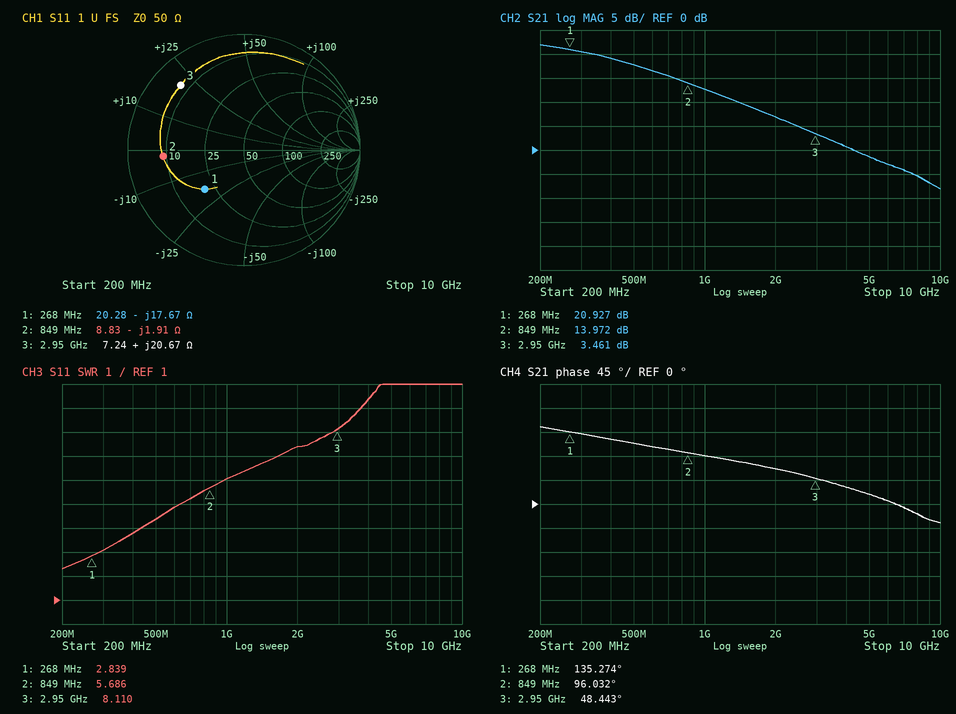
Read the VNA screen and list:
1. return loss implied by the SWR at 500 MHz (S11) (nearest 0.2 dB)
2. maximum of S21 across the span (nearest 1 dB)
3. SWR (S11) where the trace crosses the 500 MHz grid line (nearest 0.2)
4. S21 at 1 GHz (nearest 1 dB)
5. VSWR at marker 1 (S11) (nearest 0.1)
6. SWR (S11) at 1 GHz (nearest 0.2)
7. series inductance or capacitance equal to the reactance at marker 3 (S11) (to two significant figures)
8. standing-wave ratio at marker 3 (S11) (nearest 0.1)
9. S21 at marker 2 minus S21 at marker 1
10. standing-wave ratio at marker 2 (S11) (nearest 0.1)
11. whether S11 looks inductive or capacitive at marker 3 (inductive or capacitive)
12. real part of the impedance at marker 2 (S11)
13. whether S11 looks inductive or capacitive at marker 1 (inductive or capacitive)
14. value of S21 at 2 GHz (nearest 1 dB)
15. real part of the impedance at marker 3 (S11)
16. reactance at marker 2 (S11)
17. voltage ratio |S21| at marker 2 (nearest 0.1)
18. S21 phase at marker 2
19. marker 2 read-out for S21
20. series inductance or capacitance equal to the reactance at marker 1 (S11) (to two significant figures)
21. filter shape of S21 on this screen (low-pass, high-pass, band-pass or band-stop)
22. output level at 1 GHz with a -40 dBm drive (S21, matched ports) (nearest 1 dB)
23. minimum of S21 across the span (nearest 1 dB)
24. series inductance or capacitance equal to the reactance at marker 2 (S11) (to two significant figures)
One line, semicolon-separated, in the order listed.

4.0 dB; 22 dB; 4.4; 13 dB; 2.8; 6.0; 1.1 nH; 8.1; -6.955 dB; 5.7; inductive; 8.83 Ω; capacitive; 7 dB; 7.24 Ω; -1.91 Ω; 5.0; 96.032°; 13.972 dB; 34 pF; low-pass; -27 dBm; -8 dB; 98 pF
